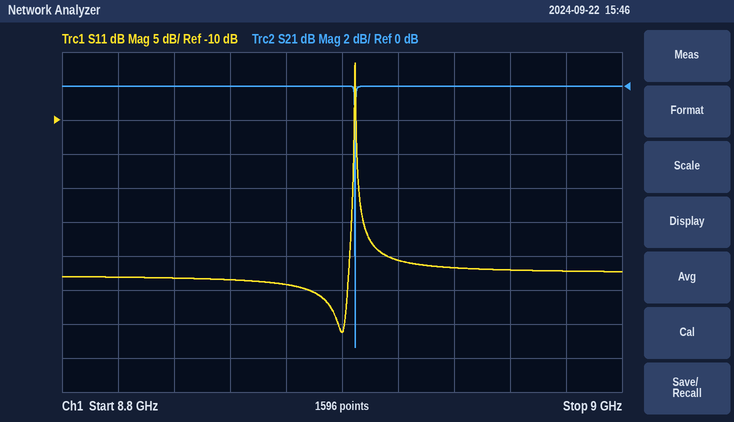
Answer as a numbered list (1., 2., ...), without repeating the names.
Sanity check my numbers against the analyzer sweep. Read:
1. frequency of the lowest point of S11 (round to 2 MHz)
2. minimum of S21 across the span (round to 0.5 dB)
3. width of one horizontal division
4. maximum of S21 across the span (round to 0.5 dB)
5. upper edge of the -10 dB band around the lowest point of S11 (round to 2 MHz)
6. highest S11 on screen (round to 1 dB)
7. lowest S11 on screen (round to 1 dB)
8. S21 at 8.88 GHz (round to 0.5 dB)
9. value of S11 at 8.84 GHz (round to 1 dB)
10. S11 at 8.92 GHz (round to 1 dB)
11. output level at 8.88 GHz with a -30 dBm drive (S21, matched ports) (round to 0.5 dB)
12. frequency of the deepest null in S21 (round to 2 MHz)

1. 8.900 GHz
2. -15.5 dB
3. 20 MHz
4. 0.0 dB
5. 8.904 GHz
6. -2 dB
7. -41 dB
8. 0.0 dB
9. -33 dB
10. -31 dB
11. -30.0 dBm
12. 8.904 GHz
